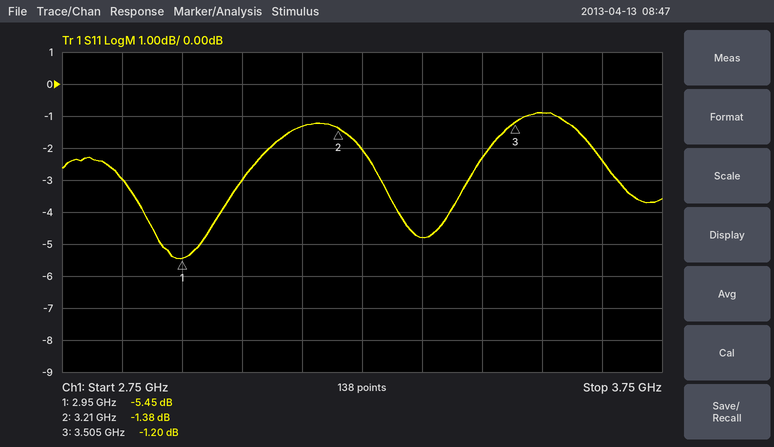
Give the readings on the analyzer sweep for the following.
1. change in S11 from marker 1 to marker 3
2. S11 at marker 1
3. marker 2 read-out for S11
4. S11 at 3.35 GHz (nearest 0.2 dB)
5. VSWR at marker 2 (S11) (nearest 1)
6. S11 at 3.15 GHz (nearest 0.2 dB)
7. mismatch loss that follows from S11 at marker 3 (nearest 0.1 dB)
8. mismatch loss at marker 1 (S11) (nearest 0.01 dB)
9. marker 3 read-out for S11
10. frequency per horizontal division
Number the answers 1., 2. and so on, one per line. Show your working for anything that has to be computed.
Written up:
1. -1.2 − (-5.45) = 4.25 dB
2. -5.45 dB
3. -1.38 dB
4. -4.8 dB
5. (1 + 0.8531)/(1 − 0.8531) ≈ 13
6. -1.4 dB
7. −10 log10(1 − 10^(-1.2/10)) ≈ 6.2 dB
8. −10 log10(1 − 10^(-5.45/10)) ≈ 1.46 dB
9. -1.20 dB
10. 100 MHz
